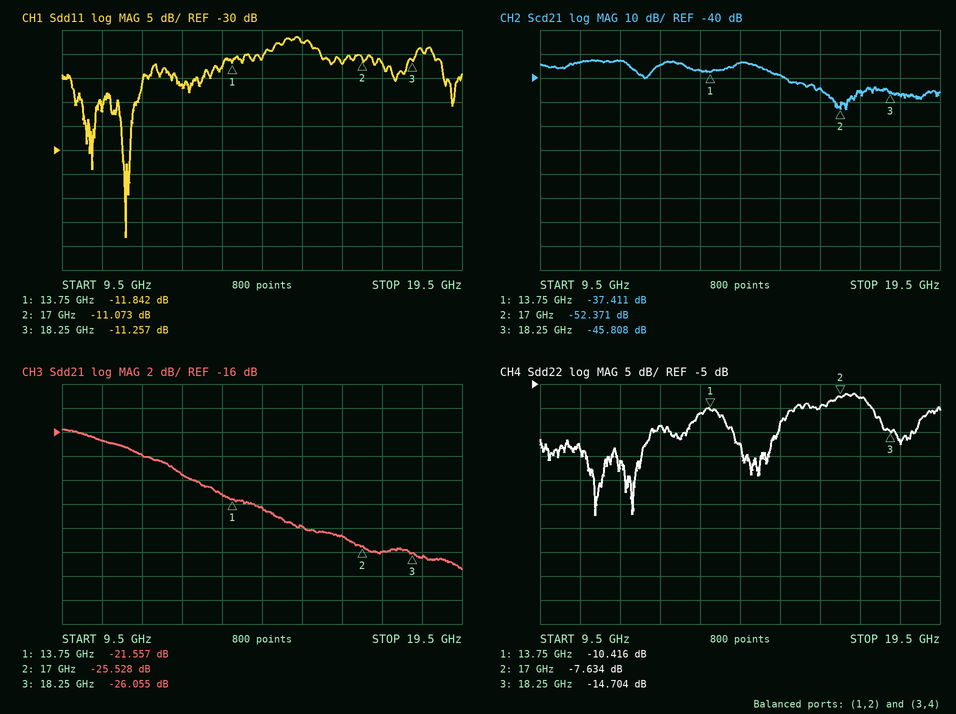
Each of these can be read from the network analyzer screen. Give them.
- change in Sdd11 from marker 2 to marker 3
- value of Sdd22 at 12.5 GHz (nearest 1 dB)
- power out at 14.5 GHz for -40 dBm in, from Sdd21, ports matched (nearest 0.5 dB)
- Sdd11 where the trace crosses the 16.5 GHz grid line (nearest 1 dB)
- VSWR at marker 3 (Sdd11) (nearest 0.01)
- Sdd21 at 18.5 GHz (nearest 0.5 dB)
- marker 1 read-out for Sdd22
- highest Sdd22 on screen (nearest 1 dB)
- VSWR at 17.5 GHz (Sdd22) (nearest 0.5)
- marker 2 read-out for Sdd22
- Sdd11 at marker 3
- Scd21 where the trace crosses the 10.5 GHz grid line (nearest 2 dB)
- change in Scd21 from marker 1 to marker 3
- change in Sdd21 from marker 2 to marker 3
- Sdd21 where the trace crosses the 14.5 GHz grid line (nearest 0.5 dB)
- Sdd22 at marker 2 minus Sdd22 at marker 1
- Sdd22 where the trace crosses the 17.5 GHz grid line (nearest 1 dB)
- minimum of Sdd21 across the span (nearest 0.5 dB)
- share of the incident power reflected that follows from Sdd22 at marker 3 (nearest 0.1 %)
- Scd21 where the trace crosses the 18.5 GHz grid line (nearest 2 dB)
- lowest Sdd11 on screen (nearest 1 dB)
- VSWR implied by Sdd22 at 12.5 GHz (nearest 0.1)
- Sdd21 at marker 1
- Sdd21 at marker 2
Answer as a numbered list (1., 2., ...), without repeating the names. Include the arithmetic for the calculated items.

1. -11.257 − (-11.073) = -0.184 dB
2. -14 dB
3. -40 dBm + (-22.5 dB) = -62.5 dBm
4. -12 dB
5. (1 + 0.2736)/(1 − 0.2736) ≈ 1.75
6. -26.5 dB
7. -10.416 dB
8. -7 dB
9. |Γ| = 10^(-8/20) = 0.3981; VSWR = (1 + 0.3981)/(1 − 0.3981) ≈ 2.32, so 2.5 to the nearest 0.5
10. -7.634 dB
11. -11.257 dB
12. -34 dB
13. -45.808 − (-37.411) = -8.397 dB
14. -26.055 − (-25.528) = -0.527 dB
15. -22.5 dB
16. -7.634 − (-10.416) = 2.782 dB
17. -8 dB
18. -27.5 dB
19. 10^(-14.704/10) ≈ 3.4 %
20. -46 dB
21. -48 dB
22. |Γ| = 10^(-14/20) = 0.1995; VSWR = (1 + 0.1995)/(1 − 0.1995) ≈ 1.5
23. -21.557 dB
24. -25.528 dB
